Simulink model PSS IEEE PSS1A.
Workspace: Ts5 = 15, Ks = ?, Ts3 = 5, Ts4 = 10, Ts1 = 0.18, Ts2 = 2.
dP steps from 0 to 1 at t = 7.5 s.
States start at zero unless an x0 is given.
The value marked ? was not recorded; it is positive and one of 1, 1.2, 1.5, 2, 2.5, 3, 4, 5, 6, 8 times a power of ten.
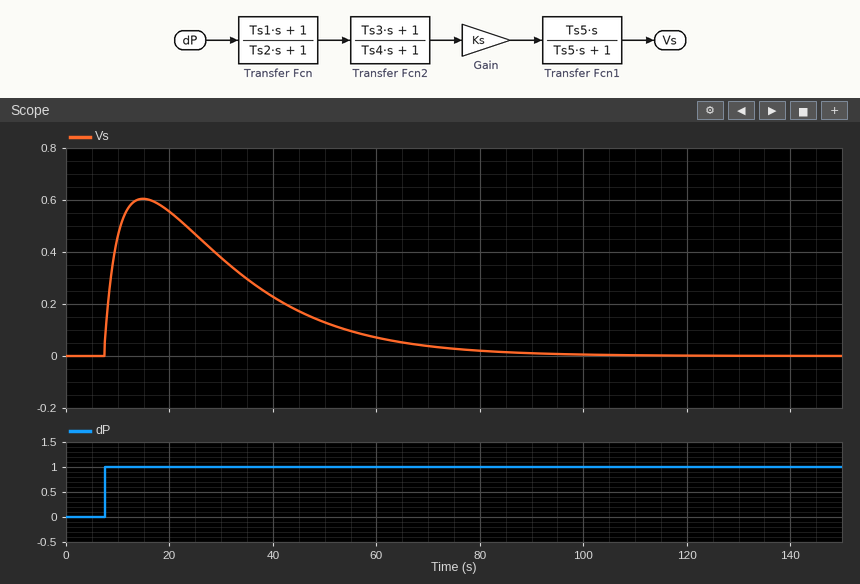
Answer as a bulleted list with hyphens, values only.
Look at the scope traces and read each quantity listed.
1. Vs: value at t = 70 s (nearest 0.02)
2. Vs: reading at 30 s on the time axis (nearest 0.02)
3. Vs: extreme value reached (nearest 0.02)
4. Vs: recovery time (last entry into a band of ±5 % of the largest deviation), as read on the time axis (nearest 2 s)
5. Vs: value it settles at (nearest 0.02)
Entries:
- 0.04
- 0.38
- 0.60
- 74 s
- 0.00
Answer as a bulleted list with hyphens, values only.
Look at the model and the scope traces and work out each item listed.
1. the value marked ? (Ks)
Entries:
- 1.2
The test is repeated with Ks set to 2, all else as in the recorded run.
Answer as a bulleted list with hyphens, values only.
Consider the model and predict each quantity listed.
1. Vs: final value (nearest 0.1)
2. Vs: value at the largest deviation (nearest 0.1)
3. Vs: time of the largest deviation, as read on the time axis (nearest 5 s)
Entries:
- 0.0
- 1.0
- 15 s
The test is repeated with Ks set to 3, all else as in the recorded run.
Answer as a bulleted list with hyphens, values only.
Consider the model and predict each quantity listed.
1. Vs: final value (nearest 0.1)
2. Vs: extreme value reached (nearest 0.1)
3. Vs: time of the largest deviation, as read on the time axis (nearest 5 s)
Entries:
- 0.0
- 1.5
- 15 s
